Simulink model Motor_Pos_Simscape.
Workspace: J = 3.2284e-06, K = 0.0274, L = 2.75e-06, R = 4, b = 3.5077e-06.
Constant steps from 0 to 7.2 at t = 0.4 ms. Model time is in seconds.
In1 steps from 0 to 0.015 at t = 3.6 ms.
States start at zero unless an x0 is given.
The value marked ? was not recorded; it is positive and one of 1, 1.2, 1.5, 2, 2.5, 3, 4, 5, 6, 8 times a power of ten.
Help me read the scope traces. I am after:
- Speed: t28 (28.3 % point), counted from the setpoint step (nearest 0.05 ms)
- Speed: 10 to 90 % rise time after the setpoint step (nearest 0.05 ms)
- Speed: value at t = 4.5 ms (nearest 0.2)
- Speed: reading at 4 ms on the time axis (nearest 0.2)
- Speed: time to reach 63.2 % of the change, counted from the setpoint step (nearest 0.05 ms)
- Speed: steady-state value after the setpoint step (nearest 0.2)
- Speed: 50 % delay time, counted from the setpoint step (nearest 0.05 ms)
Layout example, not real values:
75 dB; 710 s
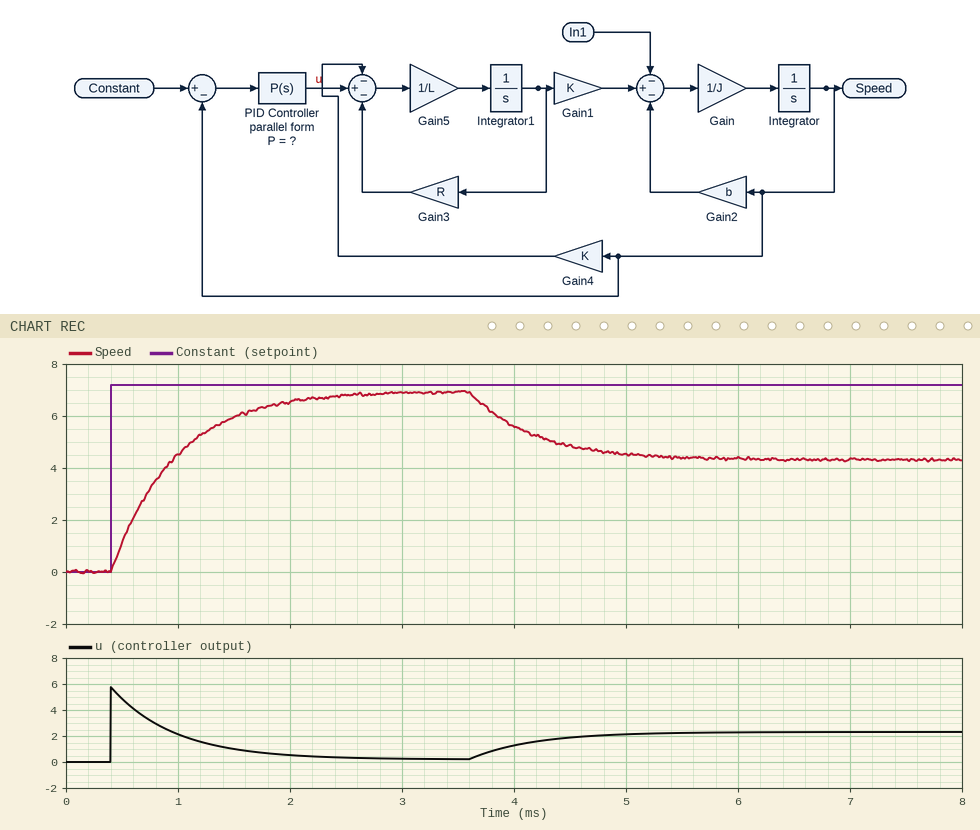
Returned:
0.20 ms; 1.25 ms; 4.8; 5.6; 0.55 ms; 7.0; 0.40 ms
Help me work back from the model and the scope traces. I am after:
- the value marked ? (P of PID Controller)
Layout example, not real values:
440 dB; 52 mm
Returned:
0.8
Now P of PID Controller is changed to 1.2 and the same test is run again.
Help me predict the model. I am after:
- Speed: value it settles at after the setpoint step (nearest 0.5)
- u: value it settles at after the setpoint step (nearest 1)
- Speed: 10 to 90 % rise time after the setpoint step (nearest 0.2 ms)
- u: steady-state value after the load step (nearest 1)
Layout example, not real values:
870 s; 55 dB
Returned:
7.0; 0; 0.8 ms; 2
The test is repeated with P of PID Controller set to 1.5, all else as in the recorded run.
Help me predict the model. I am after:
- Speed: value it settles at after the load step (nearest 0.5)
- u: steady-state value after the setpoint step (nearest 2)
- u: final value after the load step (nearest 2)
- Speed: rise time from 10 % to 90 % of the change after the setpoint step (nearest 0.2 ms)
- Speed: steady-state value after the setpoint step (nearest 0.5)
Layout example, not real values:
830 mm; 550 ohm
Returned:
5.5; 0; 2; 0.6 ms; 7.0
